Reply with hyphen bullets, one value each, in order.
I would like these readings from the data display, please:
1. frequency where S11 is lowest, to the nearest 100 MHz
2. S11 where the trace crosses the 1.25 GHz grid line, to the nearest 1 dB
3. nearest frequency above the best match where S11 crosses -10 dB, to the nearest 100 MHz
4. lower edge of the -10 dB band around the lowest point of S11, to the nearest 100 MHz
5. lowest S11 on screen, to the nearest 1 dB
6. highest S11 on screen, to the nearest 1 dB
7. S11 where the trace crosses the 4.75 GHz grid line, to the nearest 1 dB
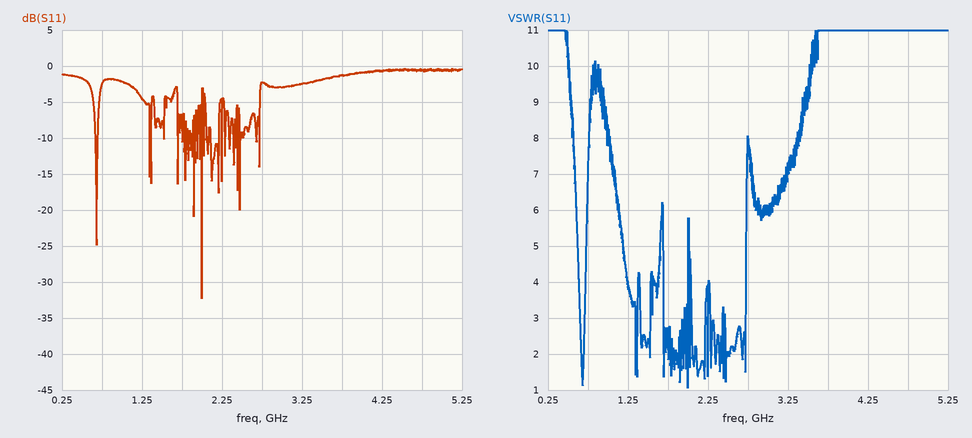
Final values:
- 2.0 GHz
- -5 dB
- 2.0 GHz
- 2.0 GHz
- -32 dB
- 0 dB
- -1 dB
